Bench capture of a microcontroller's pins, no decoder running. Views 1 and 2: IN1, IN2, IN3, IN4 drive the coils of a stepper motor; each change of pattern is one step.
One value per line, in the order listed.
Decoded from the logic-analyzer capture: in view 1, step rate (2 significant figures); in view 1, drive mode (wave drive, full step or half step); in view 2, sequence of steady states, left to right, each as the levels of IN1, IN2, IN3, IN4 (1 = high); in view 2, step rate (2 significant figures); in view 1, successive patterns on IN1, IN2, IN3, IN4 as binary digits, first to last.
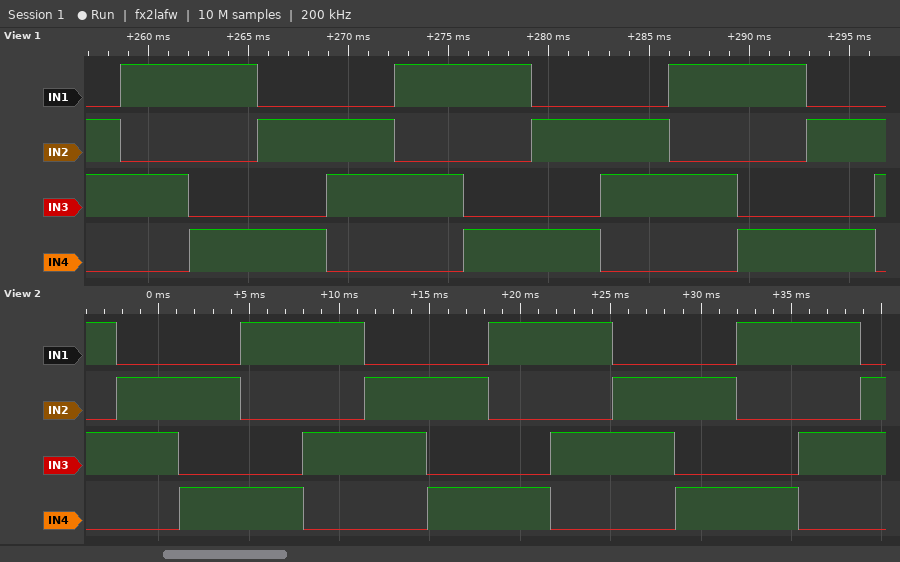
290 steps/s
full step
1010 0110 0101 1001 1010 0110 0101 1001 1010 0110 0101 1001 1010 0110
290 steps/s
0110 1010 1001 0101 0110 1010 1001 0101 0110 1010 1001 0101 0110
